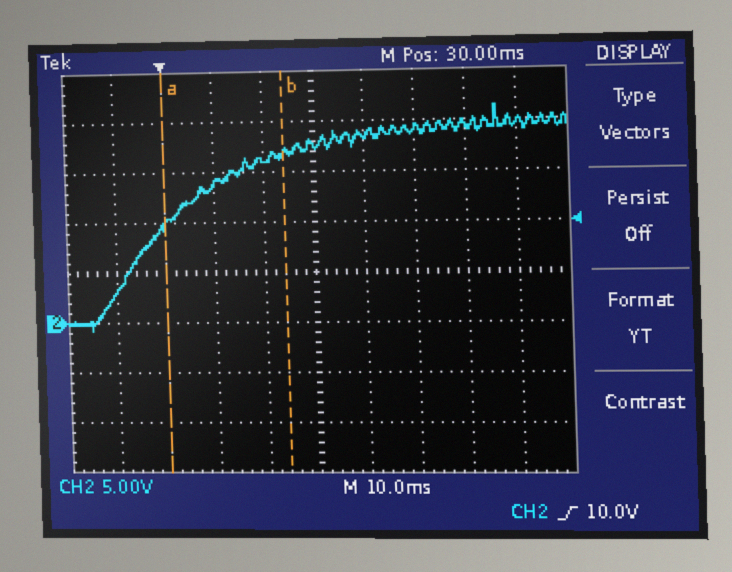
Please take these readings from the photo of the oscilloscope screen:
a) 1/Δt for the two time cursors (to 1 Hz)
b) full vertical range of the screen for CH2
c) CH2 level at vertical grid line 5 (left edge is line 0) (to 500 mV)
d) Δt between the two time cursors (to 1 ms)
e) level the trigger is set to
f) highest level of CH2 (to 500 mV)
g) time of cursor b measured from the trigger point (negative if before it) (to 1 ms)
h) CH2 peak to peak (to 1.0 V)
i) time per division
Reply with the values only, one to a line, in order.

42 Hz
40 V
17.5 V
24 ms
10.0 V
21.5 V
+24 ms
22.0 V
10 ms
